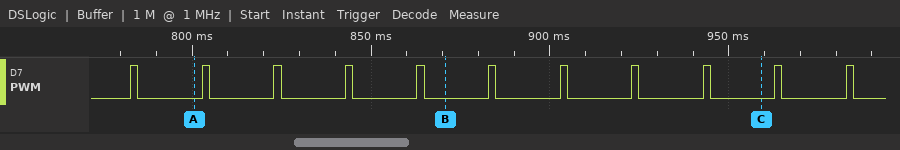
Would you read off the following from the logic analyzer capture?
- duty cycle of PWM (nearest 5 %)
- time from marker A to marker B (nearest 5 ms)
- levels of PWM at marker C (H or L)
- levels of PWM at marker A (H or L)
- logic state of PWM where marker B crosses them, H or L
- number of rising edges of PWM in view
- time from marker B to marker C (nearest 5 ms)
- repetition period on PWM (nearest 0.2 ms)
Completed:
10 %
70 ms
PWM=L
PWM=L
PWM=L
11
90 ms
20 ms
